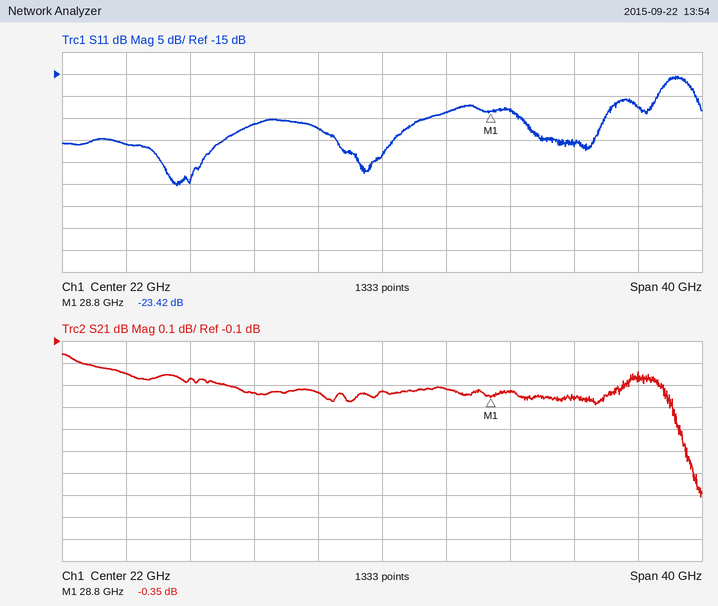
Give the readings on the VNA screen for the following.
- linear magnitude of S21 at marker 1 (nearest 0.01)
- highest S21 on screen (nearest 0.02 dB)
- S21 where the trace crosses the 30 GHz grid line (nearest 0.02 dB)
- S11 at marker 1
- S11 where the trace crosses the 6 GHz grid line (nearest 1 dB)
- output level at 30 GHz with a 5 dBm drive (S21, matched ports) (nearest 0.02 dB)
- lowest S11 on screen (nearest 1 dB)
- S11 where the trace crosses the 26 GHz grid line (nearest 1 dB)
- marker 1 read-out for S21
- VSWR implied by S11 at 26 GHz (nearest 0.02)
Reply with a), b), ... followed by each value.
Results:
a) 0.96
b) -0.16 dB
c) -0.32 dB
d) -23.42 dB
e) -31 dB
f) 4.68 dBm
g) -40 dB
h) -24 dB
i) -0.35 dB
j) 1.14
